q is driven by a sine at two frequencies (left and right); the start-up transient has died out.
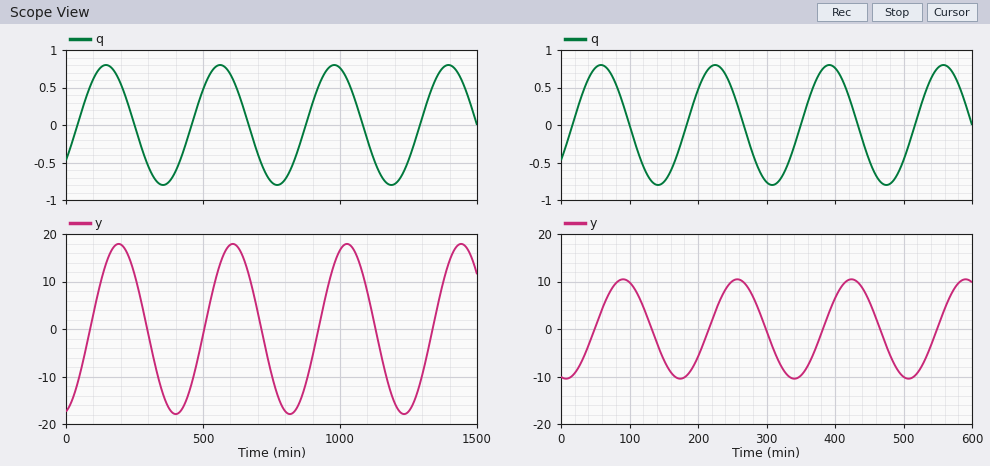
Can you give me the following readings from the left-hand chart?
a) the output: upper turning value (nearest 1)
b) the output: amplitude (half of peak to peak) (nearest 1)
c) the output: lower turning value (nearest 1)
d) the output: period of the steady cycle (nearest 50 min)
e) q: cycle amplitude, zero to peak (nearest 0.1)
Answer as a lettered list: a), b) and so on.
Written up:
a) 18
b) 18
c) -18
d) 400 min
e) 0.8
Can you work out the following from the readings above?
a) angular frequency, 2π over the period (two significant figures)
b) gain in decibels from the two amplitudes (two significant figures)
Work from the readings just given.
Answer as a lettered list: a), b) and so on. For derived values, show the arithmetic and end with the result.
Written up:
a) 2π / 400 = 0.016 rad/min
b) 20 log10(18 / 0.8) = 27 dB
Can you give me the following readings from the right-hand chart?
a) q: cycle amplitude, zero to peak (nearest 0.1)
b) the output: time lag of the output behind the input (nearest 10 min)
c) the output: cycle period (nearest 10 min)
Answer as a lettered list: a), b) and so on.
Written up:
a) 0.8
b) 30 min
c) 170 min
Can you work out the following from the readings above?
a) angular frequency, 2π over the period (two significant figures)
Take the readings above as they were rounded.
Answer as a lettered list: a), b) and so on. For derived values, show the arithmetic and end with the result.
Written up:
a) 2π / 170 = 0.037 rad/min
